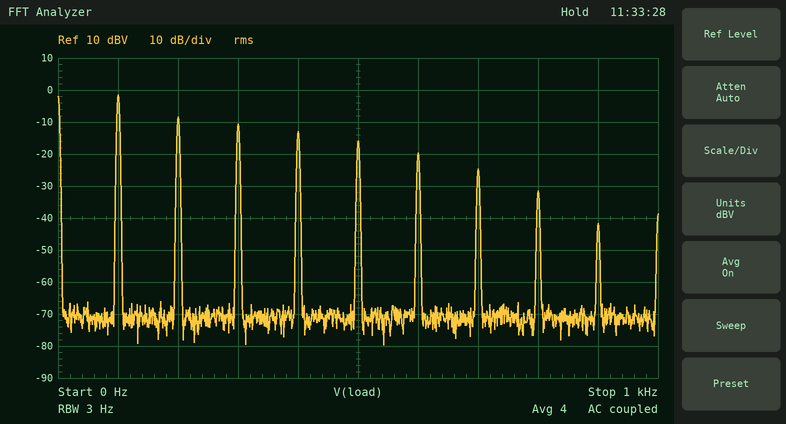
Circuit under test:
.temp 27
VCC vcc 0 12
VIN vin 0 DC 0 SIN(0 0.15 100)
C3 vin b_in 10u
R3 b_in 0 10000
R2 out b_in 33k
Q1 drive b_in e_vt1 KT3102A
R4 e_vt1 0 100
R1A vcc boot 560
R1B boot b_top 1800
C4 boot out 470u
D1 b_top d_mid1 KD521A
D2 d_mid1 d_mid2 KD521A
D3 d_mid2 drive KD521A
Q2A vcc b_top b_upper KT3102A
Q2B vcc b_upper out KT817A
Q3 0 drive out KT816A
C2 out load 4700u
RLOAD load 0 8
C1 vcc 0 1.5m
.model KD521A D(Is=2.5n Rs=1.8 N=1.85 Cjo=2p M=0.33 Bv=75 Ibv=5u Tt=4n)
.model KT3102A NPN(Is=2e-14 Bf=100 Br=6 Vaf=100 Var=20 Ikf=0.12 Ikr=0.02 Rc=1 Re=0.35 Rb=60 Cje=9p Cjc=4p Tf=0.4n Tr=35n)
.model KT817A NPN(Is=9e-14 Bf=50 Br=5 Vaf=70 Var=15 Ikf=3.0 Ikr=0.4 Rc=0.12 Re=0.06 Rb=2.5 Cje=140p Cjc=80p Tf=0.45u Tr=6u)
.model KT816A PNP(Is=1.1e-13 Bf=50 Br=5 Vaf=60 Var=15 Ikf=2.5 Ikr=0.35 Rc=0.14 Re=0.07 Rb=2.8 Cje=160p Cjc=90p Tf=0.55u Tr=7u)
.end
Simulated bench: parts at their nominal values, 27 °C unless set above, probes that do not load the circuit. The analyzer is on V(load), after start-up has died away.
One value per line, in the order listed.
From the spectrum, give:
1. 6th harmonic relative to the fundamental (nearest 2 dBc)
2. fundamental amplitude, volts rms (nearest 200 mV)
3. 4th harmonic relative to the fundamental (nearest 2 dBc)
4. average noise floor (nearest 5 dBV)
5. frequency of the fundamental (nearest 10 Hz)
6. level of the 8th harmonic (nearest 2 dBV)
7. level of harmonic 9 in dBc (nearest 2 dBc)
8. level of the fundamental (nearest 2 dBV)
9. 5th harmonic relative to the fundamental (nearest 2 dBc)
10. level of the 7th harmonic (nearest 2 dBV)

-18 dBc
800 mV
-12 dBc
-70 dBV
100 Hz
-32 dBV
-40 dBc
-2 dBV
-14 dBc
-24 dBV
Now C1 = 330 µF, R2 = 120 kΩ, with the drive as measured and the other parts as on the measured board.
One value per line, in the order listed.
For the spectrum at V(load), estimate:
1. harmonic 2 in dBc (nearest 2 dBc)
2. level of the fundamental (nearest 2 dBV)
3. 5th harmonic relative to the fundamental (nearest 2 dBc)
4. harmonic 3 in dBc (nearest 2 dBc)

-12 dBc
-4 dBV
-20 dBc
-18 dBc
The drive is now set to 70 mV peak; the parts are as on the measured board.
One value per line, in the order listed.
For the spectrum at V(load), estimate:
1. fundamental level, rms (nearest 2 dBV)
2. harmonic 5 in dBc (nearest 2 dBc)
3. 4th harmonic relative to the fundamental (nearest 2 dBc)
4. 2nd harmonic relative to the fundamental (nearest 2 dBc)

-10 dBV
-32 dBc
-26 dBc
-14 dBc
